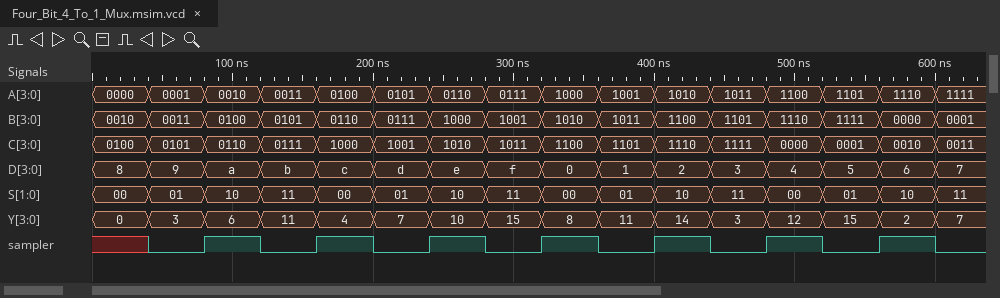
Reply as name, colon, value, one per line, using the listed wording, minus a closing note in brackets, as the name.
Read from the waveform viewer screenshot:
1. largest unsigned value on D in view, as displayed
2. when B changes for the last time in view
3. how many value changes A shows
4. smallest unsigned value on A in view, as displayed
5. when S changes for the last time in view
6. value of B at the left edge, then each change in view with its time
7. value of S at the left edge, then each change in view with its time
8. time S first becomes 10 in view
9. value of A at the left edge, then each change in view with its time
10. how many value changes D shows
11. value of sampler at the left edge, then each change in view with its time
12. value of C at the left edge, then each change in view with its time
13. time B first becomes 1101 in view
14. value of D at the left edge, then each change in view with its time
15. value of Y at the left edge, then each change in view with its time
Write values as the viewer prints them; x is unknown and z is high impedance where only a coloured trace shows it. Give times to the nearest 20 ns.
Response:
largest unsigned value on D in view, as displayed: f
when B changes for the last time in view: 600 ns
how many value changes A shows: 15
smallest unsigned value on A in view, as displayed: 0000
when S changes for the last time in view: 600 ns
value of B at the left edge, then each change in view with its time: 0010, 0011 at 40 ns, 0100 at 80 ns, 0101 at 120 ns, 0110 at 160 ns, 0111 at 200 ns, 1000 at 240 ns, 1001 at 280 ns, 1010 at 320 ns, 1011 at 360 ns, 1100 at 400 ns, 1101 at 440 ns, 1110 at 480 ns, 1111 at 520 ns, 0000 at 560 ns, 0001 at 600 ns
value of S at the left edge, then each change in view with its time: 00, 01 at 40 ns, 10 at 80 ns, 11 at 120 ns, 00 at 160 ns, 01 at 200 ns, 10 at 240 ns, 11 at 280 ns, 00 at 320 ns, 01 at 360 ns, 10 at 400 ns, 11 at 440 ns, 00 at 480 ns, 01 at 520 ns, 10 at 560 ns, 11 at 600 ns
time S first becomes 10 in view: 80 ns
value of A at the left edge, then each change in view with its time: 0000, 0001 at 40 ns, 0010 at 80 ns, 0011 at 120 ns, 0100 at 160 ns, 0101 at 200 ns, 0110 at 240 ns, 0111 at 280 ns, 1000 at 320 ns, 1001 at 360 ns, 1010 at 400 ns, 1011 at 440 ns, 1100 at 480 ns, 1101 at 520 ns, 1110 at 560 ns, 1111 at 600 ns
how many value changes D shows: 15
value of sampler at the left edge, then each change in view with its time: x, 0 at 40 ns, 1 at 80 ns, 0 at 120 ns, 1 at 160 ns, 0 at 200 ns, 1 at 240 ns, 0 at 280 ns, 1 at 320 ns, 0 at 360 ns, 1 at 400 ns, 0 at 440 ns, 1 at 480 ns, 0 at 520 ns, 1 at 560 ns, 0 at 600 ns
value of C at the left edge, then each change in view with its time: 0100, 0101 at 40 ns, 0110 at 80 ns, 0111 at 120 ns, 1000 at 160 ns, 1001 at 200 ns, 1010 at 240 ns, 1011 at 280 ns, 1100 at 320 ns, 1101 at 360 ns, 1110 at 400 ns, 1111 at 440 ns, 0000 at 480 ns, 0001 at 520 ns, 0010 at 560 ns, 0011 at 600 ns
time B first becomes 1101 in view: 440 ns
value of D at the left edge, then each change in view with its time: 8, 9 at 40 ns, a at 80 ns, b at 120 ns, c at 160 ns, d at 200 ns, e at 240 ns, f at 280 ns, 0 at 320 ns, 1 at 360 ns, 2 at 400 ns, 3 at 440 ns, 4 at 480 ns, 5 at 520 ns, 6 at 560 ns, 7 at 600 ns
value of Y at the left edge, then each change in view with its time: 0, 3 at 40 ns, 6 at 80 ns, 11 at 120 ns, 4 at 160 ns, 7 at 200 ns, 10 at 240 ns, 15 at 280 ns, 8 at 320 ns, 11 at 360 ns, 14 at 400 ns, 3 at 440 ns, 12 at 480 ns, 15 at 520 ns, 2 at 560 ns, 7 at 600 ns
